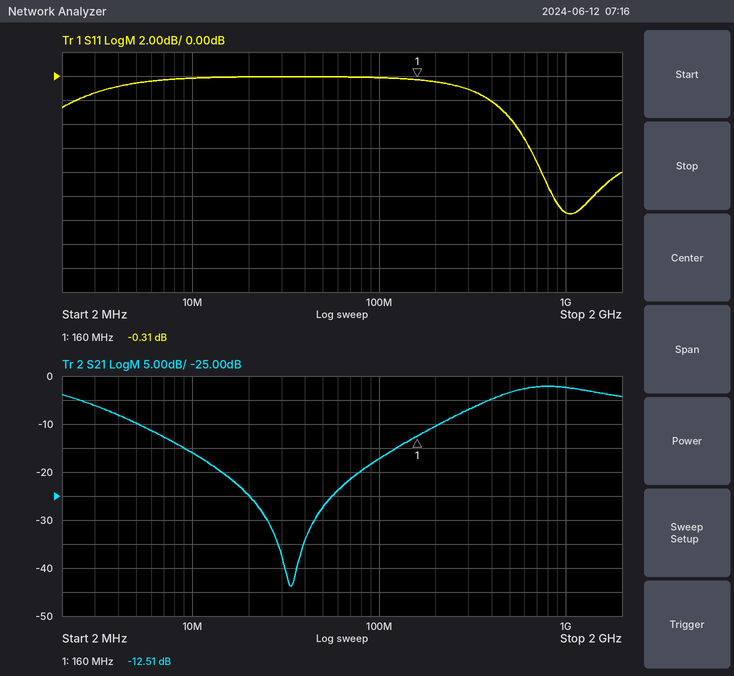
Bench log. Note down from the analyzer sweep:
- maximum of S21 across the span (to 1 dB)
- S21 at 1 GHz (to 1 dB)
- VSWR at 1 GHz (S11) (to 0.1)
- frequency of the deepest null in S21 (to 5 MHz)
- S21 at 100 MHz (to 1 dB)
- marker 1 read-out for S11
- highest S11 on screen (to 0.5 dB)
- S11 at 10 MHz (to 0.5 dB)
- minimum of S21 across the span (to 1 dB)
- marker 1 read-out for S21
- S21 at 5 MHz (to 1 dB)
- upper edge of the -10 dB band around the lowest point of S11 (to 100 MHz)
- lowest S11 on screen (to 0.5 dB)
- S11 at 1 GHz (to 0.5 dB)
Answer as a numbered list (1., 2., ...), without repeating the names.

1. -2 dB
2. -2 dB
3. 1.7
4. 35 MHz
5. -17 dB
6. -0.31 dB
7. 0.0 dB
8. 0.0 dB
9. -44 dB
10. -12.51 dB
11. -10 dB
12. 1.4 GHz
13. -11.5 dB
14. -11.5 dB
